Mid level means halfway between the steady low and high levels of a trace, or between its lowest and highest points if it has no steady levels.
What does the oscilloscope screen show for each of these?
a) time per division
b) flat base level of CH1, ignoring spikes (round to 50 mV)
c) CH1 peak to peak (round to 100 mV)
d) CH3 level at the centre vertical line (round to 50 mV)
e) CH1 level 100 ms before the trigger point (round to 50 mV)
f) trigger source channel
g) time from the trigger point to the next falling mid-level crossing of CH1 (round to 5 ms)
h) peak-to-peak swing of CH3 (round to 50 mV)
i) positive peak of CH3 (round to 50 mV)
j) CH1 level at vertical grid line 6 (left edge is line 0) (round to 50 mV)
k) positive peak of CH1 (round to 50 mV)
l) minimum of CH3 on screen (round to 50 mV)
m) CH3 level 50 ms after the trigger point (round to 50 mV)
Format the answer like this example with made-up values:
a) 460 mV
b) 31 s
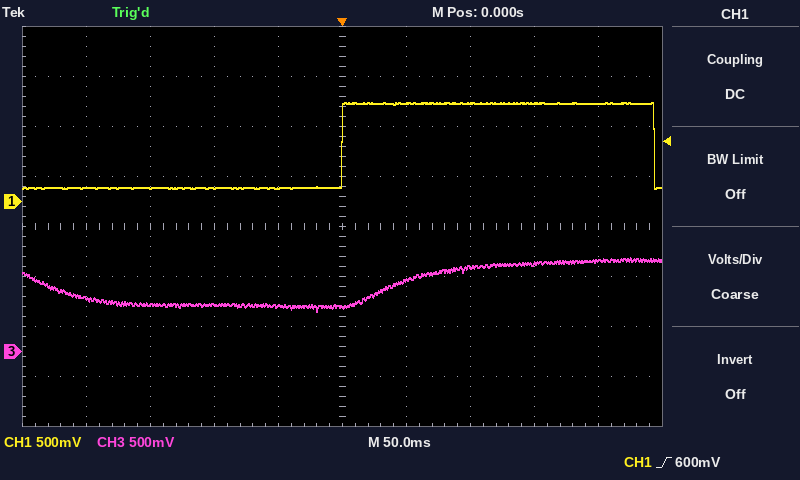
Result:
a) 50 ms
b) 150 mV
c) 900 mV
d) 450 mV
e) 150 mV
f) CH1
g) 245 ms
h) 550 mV
i) 950 mV
j) 1.00 V
k) 1.00 V
l) 400 mV
m) 700 mV
